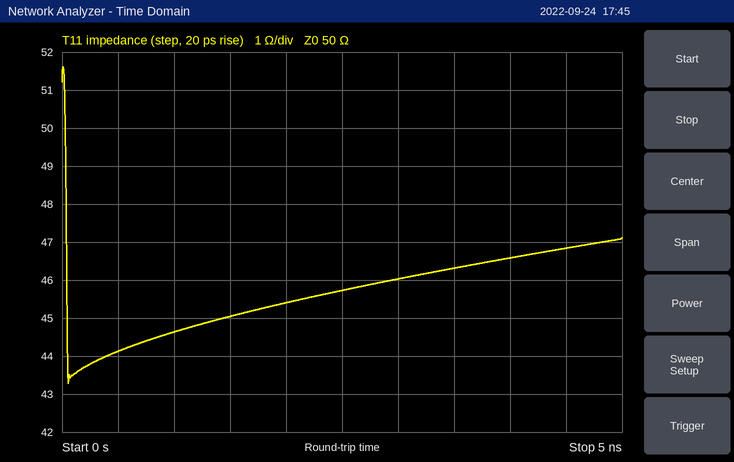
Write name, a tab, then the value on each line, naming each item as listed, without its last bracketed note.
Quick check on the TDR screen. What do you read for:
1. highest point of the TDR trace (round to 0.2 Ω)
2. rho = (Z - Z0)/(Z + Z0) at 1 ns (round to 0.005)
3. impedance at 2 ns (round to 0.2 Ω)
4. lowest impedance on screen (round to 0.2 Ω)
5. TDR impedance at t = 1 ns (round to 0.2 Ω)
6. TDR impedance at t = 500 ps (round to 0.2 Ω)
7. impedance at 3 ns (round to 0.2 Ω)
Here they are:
highest point of the TDR trace	51.6 Ω
rho = (Z - Z0)/(Z + Z0) at 1 ns	-0.055
impedance at 2 ns	45.4 Ω
lowest impedance on screen	43.2 Ω
TDR impedance at t = 1 ns	44.6 Ω
TDR impedance at t = 500 ps	44.2 Ω
impedance at 3 ns	46.0 Ω
